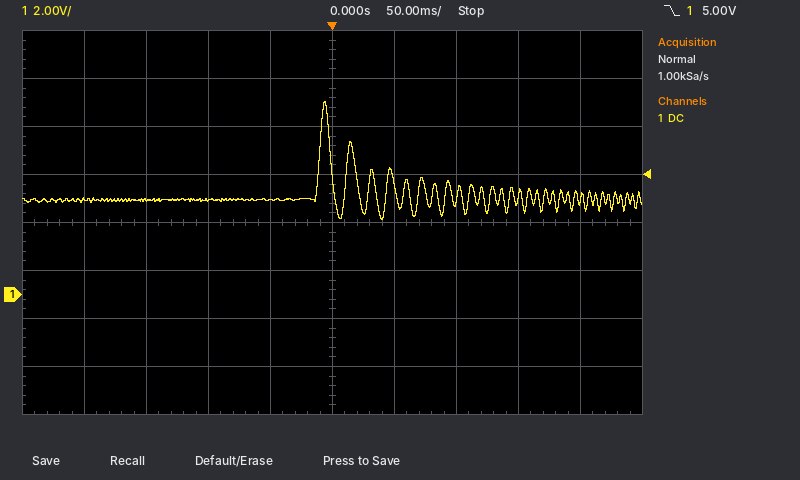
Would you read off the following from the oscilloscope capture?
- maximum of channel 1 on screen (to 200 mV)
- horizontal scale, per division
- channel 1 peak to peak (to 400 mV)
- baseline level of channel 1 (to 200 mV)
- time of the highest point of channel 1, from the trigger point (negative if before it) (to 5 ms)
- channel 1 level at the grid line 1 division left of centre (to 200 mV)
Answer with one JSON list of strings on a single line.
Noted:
["8.0 V", "50 ms", "4.8 V", "4.0 V", "-5 ms", "4.0 V"]
